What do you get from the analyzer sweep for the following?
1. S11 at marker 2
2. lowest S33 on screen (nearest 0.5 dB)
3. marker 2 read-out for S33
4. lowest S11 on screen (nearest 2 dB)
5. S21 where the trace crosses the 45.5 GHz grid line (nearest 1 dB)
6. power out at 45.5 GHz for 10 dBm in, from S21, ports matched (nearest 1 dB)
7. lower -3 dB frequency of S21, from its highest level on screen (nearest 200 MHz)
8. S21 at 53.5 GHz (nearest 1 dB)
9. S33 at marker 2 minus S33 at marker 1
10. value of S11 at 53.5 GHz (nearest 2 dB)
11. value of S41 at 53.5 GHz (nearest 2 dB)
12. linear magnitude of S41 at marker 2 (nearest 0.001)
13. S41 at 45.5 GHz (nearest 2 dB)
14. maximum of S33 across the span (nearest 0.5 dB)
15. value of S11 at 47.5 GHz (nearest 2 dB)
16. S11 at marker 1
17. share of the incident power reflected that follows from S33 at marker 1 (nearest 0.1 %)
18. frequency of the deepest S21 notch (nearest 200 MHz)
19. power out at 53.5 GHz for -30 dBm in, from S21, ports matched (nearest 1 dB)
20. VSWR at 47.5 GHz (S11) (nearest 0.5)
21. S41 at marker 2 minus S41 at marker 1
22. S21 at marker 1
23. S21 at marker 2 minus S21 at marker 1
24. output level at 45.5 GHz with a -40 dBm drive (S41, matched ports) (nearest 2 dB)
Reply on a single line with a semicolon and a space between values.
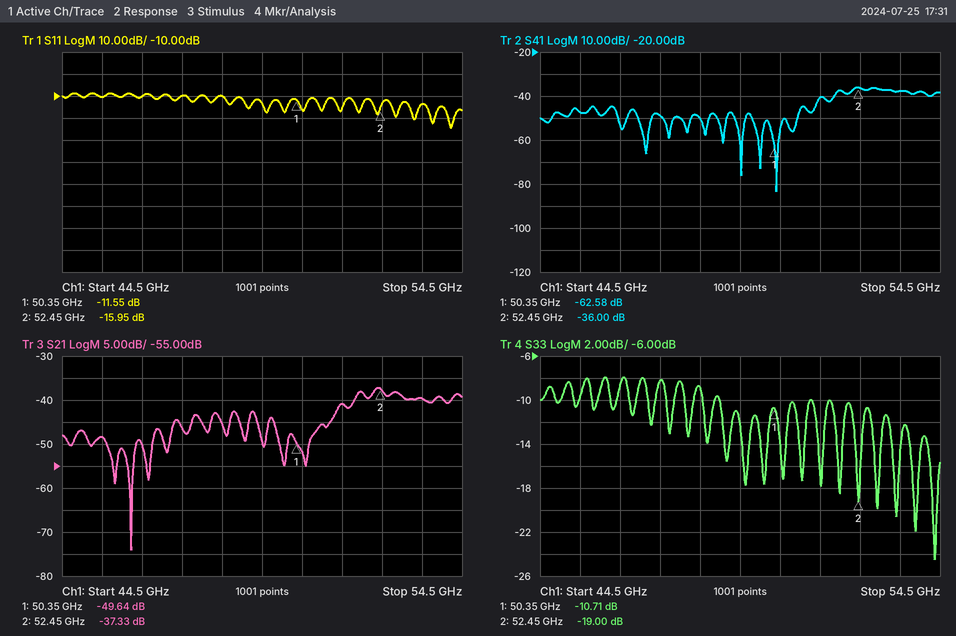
-15.95 dB; -24.5 dB; -19.00 dB; -24 dB; -48 dB; -38 dBm; 51.8 GHz; -40 dB; -8.29 dB; -14 dB; -38 dB; 0.016; -48 dB; -8.0 dB; -10 dB; -11.55 dB; 8.5 %; 46.2 GHz; -70 dBm; 2.0; 26.58 dB; -49.64 dB; 12.31 dB; -88 dBm
